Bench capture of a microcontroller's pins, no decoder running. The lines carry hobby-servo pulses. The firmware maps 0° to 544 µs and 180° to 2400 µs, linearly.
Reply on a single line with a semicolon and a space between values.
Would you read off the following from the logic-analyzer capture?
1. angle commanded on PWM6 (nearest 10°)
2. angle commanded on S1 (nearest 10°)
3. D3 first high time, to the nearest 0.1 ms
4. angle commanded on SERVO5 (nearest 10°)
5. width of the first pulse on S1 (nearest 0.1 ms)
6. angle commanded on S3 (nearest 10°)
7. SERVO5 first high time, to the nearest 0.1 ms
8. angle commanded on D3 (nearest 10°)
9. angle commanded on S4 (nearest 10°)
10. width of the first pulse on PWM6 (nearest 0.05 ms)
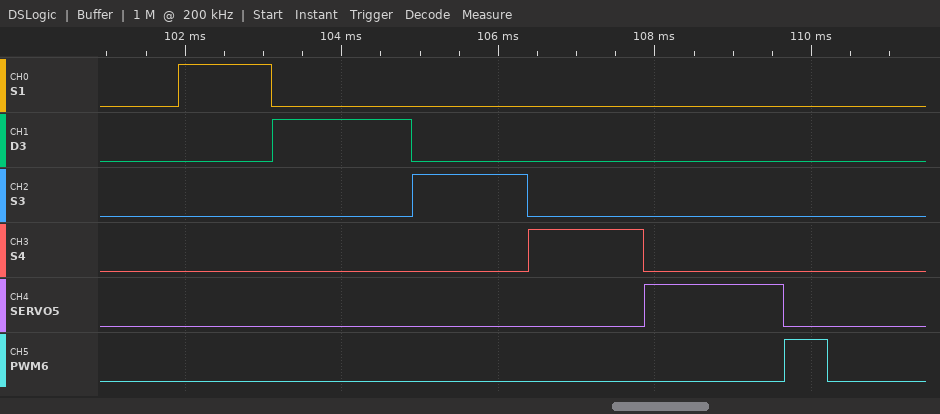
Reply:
0°; 60°; 1.8 ms; 120°; 1.2 ms; 90°; 1.8 ms; 120°; 90°; 0.55 ms
